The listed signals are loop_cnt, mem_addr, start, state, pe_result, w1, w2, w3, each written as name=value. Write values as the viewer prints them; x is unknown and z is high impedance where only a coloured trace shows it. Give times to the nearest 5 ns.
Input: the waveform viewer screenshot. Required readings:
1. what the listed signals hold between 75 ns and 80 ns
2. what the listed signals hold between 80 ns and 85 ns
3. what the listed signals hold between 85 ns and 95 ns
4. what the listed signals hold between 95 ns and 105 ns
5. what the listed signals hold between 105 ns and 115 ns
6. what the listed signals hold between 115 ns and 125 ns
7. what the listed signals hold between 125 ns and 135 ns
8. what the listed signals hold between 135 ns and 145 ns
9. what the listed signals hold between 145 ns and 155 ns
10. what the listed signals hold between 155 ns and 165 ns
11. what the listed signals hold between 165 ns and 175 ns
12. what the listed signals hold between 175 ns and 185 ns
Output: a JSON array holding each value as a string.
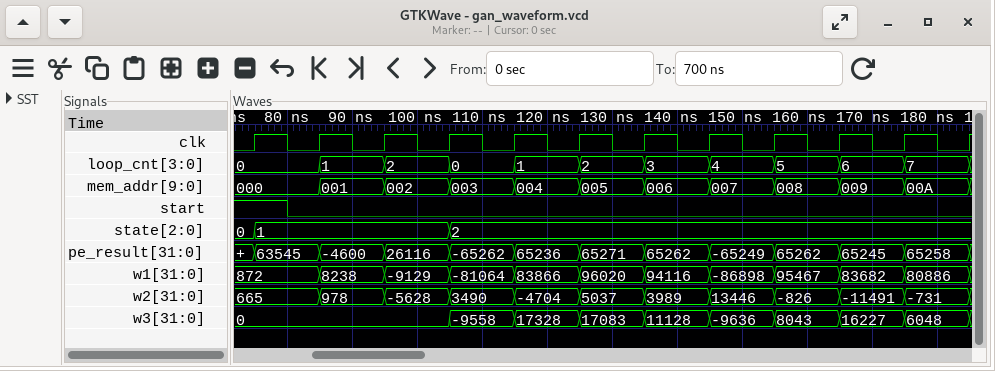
["loop_cnt=0, mem_addr=000, start=1, state=1, pe_result=63545, w1=872, w2=665, w3=0", "loop_cnt=0, mem_addr=000, start=0, state=1, pe_result=63545, w1=872, w2=665, w3=0", "loop_cnt=1, mem_addr=001, start=0, state=1, pe_result=-4600, w1=8238, w2=978, w3=0", "loop_cnt=2, mem_addr=002, start=0, state=1, pe_result=26116, w1=-9129, w2=-5628, w3=0", "loop_cnt=0, mem_addr=003, start=0, state=2, pe_result=-65262, w1=-81064, w2=3490, w3=-9558", "loop_cnt=1, mem_addr=004, start=0, state=2, pe_result=65236, w1=83866, w2=-4704, w3=17328", "loop_cnt=2, mem_addr=005, start=0, state=2, pe_result=65271, w1=96020, w2=5037, w3=17083", "loop_cnt=3, mem_addr=006, start=0, state=2, pe_result=65262, w1=94116, w2=3989, w3=11128", "loop_cnt=4, mem_addr=007, start=0, state=2, pe_result=-65249, w1=-86898, w2=13446, w3=-9636", "loop_cnt=5, mem_addr=008, start=0, state=2, pe_result=65262, w1=95467, w2=-826, w3=8043", "loop_cnt=6, mem_addr=009, start=0, state=2, pe_result=65245, w1=83682, w2=-11491, w3=16227", "loop_cnt=7, mem_addr=00A, start=0, state=2, pe_result=65258, w1=80886, w2=-731, w3=6048"]
